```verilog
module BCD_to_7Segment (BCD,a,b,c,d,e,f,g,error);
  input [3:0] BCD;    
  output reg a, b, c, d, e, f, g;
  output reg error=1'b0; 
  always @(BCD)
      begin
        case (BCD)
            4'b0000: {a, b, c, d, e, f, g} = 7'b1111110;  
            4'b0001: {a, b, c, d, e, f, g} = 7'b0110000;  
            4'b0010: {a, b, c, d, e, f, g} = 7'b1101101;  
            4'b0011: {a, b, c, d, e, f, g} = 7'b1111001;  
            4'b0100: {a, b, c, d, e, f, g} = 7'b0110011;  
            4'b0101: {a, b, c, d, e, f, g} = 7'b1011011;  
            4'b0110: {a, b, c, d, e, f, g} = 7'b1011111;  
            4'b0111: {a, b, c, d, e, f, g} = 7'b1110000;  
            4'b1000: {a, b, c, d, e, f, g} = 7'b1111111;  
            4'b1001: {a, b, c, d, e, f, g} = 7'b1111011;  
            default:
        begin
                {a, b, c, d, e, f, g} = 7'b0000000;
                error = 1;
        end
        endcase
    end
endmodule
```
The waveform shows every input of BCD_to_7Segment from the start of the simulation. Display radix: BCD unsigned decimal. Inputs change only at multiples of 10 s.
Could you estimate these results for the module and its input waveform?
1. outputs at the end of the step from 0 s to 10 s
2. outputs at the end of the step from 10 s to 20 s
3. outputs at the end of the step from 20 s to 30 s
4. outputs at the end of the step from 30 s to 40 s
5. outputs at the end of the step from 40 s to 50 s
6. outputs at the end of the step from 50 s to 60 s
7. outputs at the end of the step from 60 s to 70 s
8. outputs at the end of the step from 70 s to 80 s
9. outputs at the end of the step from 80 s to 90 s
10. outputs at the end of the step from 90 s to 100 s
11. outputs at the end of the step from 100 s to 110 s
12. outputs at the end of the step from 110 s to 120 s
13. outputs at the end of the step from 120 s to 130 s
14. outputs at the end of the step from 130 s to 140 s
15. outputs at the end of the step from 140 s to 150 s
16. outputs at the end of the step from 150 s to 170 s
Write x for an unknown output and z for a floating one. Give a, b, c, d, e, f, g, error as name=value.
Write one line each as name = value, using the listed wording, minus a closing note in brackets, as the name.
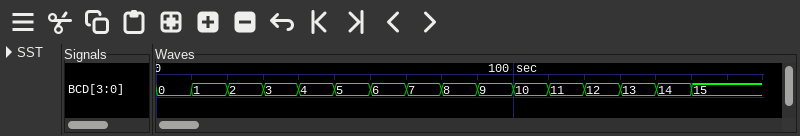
outputs at the end of the step from 0 s to 10 s = a=1, b=1, c=1, d=1, e=1, f=1, g=0, error=0
outputs at the end of the step from 10 s to 20 s = a=0, b=1, c=1, d=0, e=0, f=0, g=0, error=0
outputs at the end of the step from 20 s to 30 s = a=1, b=1, c=0, d=1, e=1, f=0, g=1, error=0
outputs at the end of the step from 30 s to 40 s = a=1, b=1, c=1, d=1, e=0, f=0, g=1, error=0
outputs at the end of the step from 40 s to 50 s = a=0, b=1, c=1, d=0, e=0, f=1, g=1, error=0
outputs at the end of the step from 50 s to 60 s = a=1, b=0, c=1, d=1, e=0, f=1, g=1, error=0
outputs at the end of the step from 60 s to 70 s = a=1, b=0, c=1, d=1, e=1, f=1, g=1, error=0
outputs at the end of the step from 70 s to 80 s = a=1, b=1, c=1, d=0, e=0, f=0, g=0, error=0
outputs at the end of the step from 80 s to 90 s = a=1, b=1, c=1, d=1, e=1, f=1, g=1, error=0
outputs at the end of the step from 90 s to 100 s = a=1, b=1, c=1, d=1, e=0, f=1, g=1, error=0
outputs at the end of the step from 100 s to 110 s = a=0, b=0, c=0, d=0, e=0, f=0, g=0, error=1
outputs at the end of the step from 110 s to 120 s = a=0, b=0, c=0, d=0, e=0, f=0, g=0, error=1
outputs at the end of the step from 120 s to 130 s = a=0, b=0, c=0, d=0, e=0, f=0, g=0, error=1
outputs at the end of the step from 130 s to 140 s = a=0, b=0, c=0, d=0, e=0, f=0, g=0, error=1
outputs at the end of the step from 140 s to 150 s = a=0, b=0, c=0, d=0, e=0, f=0, g=0, error=1
outputs at the end of the step from 150 s to 170 s = a=0, b=0, c=0, d=0, e=0, f=0, g=0, error=1
